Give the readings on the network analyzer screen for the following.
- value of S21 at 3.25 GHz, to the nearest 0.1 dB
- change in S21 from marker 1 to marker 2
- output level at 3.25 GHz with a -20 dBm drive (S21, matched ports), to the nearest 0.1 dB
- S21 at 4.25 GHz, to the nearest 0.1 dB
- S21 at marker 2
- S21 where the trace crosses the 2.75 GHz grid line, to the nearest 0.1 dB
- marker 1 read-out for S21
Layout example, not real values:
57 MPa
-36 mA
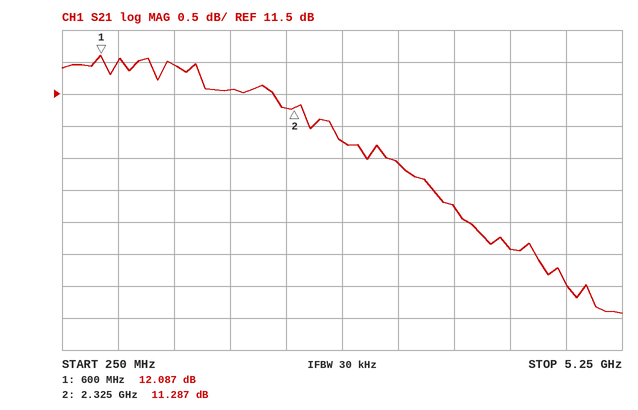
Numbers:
10.4 dB
-0.800 dB
-9.6 dBm
9.1 dB
11.287 dB
10.8 dB
12.087 dB
